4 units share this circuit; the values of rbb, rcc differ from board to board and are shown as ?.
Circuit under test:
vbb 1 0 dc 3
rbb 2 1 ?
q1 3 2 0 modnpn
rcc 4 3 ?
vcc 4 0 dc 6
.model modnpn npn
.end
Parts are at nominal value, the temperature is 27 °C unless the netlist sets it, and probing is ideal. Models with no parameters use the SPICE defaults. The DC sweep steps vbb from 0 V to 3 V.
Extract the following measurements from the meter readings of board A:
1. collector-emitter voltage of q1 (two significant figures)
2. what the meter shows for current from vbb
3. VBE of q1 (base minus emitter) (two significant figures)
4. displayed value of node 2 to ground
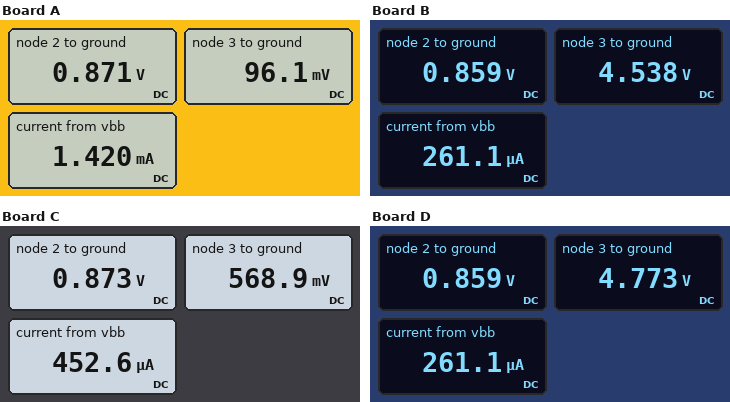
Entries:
96 mV
1.420 mA
870 mV
0.871 V
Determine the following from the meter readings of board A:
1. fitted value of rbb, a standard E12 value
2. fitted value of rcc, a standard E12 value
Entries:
1.5 kΩ
150 Ω
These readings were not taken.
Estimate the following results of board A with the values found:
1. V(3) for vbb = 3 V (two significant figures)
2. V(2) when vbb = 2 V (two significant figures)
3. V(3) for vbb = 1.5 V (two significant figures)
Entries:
96 mV
870 mV
180 mV
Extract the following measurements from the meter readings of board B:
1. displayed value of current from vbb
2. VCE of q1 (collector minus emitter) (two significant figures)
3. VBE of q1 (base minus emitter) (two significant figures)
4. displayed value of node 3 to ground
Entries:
261.1 µA
4.5 V
860 mV
4.538 V
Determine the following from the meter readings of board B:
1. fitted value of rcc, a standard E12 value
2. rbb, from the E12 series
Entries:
56 Ω
8.2 kΩ
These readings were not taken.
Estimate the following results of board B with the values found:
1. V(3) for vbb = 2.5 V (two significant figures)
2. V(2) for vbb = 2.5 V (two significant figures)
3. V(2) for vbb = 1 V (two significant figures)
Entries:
4.9 V
850 mV
800 mV
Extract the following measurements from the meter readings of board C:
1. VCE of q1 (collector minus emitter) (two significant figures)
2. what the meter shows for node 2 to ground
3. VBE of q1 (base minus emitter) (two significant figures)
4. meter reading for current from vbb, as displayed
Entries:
570 mV
0.873 V
870 mV
452.6 µA
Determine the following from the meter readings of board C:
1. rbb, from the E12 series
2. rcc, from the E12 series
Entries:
4.7 kΩ
120 Ω
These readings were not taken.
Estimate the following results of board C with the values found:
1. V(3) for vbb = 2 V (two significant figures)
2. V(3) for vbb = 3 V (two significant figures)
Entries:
3.1 V
570 mV
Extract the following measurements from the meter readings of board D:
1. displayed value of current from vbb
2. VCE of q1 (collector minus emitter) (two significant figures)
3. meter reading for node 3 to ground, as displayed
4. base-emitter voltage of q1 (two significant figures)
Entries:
261.1 µA
4.8 V
4.773 V
860 mV
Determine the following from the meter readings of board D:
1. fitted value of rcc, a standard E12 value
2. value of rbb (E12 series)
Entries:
47 Ω
8.2 kΩ
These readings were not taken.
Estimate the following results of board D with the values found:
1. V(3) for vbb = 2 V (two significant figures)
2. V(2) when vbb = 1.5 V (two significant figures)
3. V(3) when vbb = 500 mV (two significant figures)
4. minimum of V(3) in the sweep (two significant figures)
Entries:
5.3 V
830 mV
6.0 V
4.8 V
